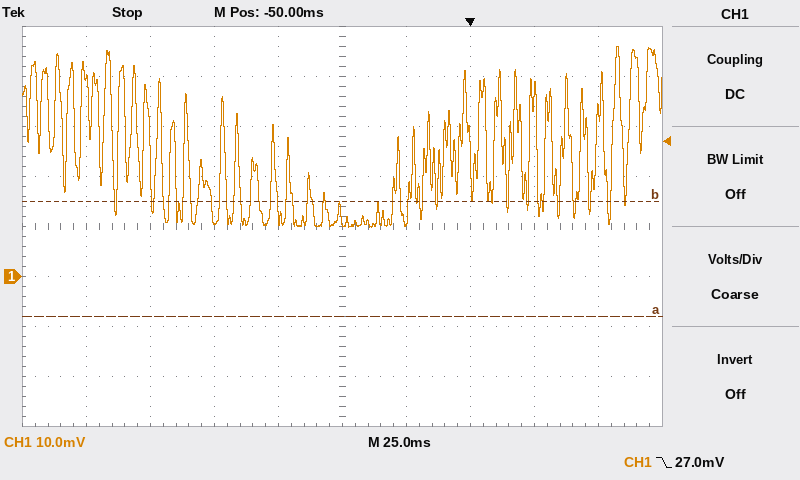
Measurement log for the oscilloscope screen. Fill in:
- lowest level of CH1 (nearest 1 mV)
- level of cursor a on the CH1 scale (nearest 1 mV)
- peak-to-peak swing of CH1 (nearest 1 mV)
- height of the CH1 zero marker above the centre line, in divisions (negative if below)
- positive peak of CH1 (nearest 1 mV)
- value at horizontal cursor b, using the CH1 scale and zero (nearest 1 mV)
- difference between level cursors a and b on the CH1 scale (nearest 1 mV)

10 mV
-8 mV
36 mV
-1.0 div
46 mV
15 mV
23 mV
